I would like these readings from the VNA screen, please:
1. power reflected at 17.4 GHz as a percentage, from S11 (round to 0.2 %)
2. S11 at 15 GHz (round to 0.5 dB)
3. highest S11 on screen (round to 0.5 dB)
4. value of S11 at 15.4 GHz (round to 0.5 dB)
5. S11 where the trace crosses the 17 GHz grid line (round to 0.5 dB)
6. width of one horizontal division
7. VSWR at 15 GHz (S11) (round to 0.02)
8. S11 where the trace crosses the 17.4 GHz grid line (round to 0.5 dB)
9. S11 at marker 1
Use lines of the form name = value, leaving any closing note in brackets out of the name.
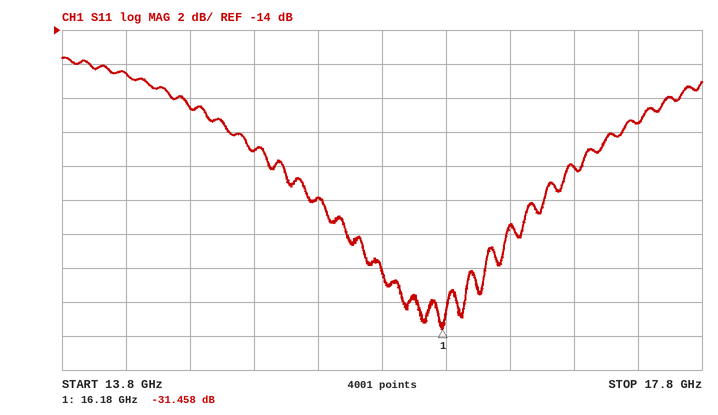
power reflected at 17.4 GHz as a percentage, from S11 = 1.2 %
S11 at 15 GHz = -21.0 dB
highest S11 on screen = -15.5 dB
value of S11 at 15.4 GHz = -24.0 dB
S11 where the trace crosses the 17 GHz grid line = -22.0 dB
width of one horizontal division = 400 MHz
VSWR at 15 GHz (S11) = 1.20
S11 where the trace crosses the 17.4 GHz grid line = -19.5 dB
S11 at marker 1 = -31.458 dB
